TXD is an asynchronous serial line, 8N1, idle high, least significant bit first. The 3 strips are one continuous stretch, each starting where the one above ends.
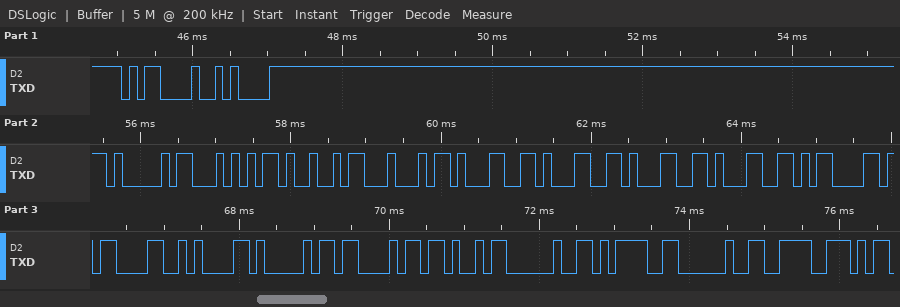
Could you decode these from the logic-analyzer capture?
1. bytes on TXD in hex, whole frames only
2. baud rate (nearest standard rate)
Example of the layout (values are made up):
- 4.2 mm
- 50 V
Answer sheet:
- 0x0D 0x0A 0x41 0x54 0x49 0x44 0x31 0x31 0x31 0x31 0x0D 0x0D 0x0A 0x41 0x43 0x4B 0x20 0x3D 0x20 0x9E
- 9600 baud
